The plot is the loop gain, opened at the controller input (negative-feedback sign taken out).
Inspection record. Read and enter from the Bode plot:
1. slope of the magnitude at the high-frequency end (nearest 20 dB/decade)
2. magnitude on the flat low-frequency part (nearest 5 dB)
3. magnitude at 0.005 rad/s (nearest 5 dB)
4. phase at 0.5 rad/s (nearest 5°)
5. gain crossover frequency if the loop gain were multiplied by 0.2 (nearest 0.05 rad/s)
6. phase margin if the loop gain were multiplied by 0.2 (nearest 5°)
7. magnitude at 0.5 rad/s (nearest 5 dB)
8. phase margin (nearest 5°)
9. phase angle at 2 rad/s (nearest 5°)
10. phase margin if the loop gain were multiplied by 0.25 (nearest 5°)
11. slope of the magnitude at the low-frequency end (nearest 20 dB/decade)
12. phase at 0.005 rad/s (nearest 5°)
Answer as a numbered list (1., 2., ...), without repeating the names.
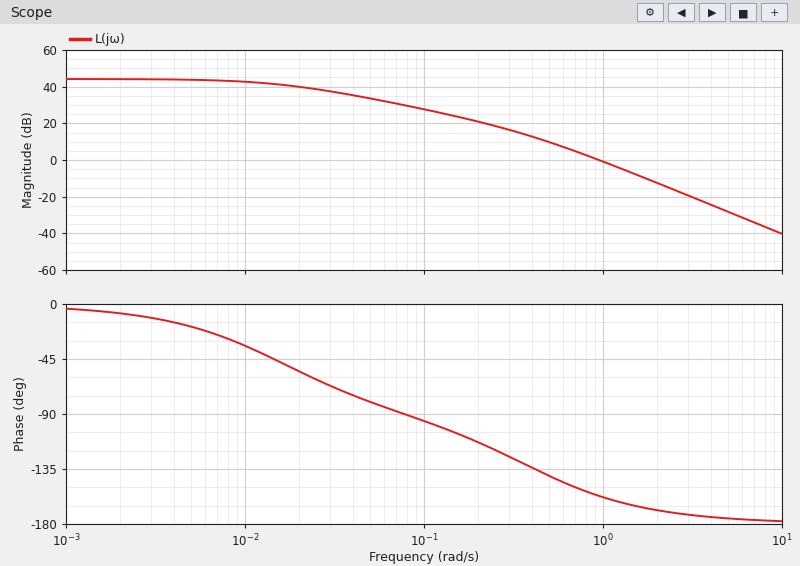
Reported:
1. -40 dB/decade
2. 45 dB
3. 45 dB
4. -140°
5. 0.35 rad/s
6. 50°
7. 10 dB
8. 25°
9. -170°
10. 45°
11. 0 dB/decade
12. -20°
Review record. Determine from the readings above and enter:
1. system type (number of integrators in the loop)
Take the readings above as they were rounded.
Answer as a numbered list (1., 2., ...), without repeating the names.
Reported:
1. 0
